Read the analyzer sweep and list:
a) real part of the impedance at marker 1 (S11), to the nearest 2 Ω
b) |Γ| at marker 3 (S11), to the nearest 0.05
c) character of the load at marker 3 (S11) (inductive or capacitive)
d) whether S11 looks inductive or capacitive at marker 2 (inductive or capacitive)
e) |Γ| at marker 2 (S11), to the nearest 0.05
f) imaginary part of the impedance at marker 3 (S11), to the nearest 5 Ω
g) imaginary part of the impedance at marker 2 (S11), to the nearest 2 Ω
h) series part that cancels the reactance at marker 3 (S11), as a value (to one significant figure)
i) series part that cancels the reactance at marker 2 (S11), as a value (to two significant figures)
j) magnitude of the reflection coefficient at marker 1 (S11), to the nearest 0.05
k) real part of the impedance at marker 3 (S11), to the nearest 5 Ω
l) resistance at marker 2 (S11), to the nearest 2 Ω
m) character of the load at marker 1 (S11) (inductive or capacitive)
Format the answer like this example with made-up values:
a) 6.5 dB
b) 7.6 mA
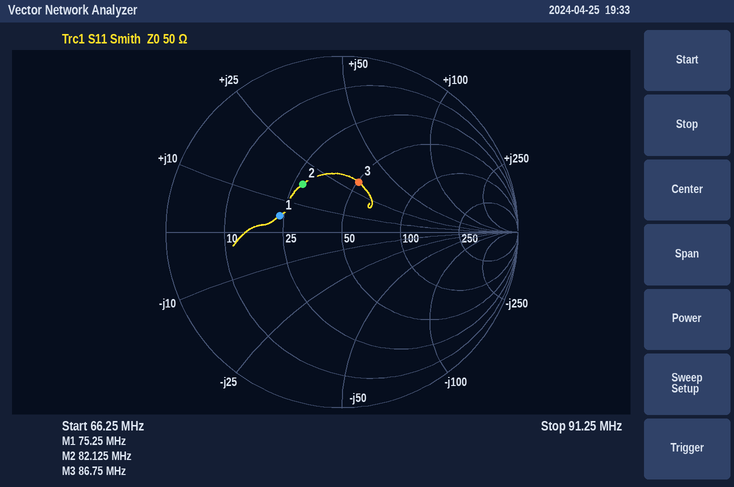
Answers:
a) 24 Ω
b) 0.30
c) inductive
d) inductive
e) 0.35
f) +30 Ω
g) +18 Ω
h) 60 pF
i) 110 pF
j) 0.35
k) 50 Ω
l) 28 Ω
m) inductive
